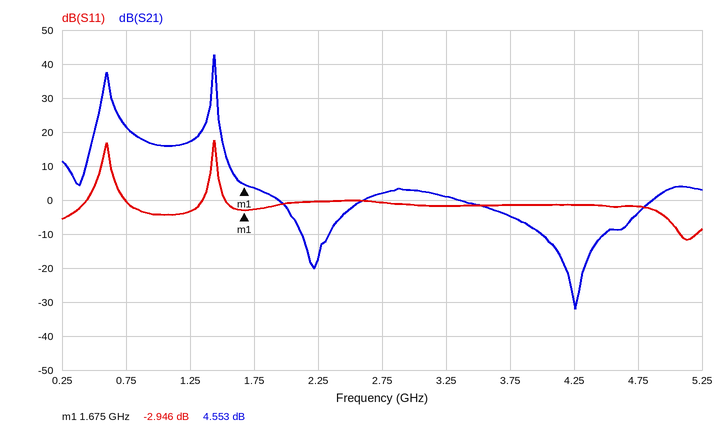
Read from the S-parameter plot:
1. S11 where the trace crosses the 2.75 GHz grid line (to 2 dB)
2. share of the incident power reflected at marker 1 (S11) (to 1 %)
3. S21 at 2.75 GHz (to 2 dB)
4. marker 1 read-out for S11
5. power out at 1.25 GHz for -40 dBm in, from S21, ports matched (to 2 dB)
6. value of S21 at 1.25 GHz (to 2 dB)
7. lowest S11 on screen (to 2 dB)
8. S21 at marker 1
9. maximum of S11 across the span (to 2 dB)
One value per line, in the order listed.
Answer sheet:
0 dB
51 %
2 dB
-2.946 dB
-22 dBm
18 dB
-12 dB
4.553 dB
18 dB
